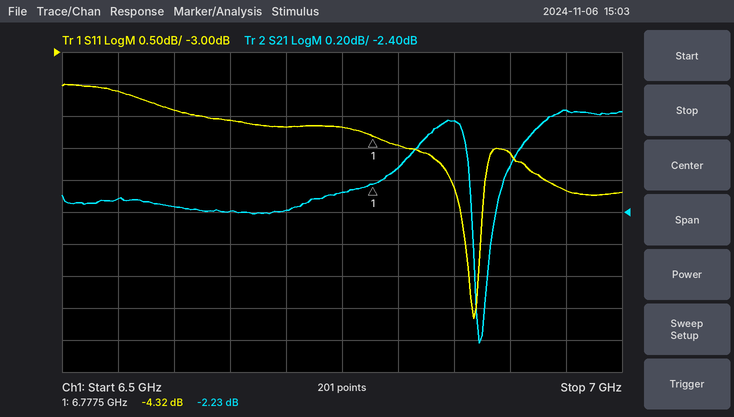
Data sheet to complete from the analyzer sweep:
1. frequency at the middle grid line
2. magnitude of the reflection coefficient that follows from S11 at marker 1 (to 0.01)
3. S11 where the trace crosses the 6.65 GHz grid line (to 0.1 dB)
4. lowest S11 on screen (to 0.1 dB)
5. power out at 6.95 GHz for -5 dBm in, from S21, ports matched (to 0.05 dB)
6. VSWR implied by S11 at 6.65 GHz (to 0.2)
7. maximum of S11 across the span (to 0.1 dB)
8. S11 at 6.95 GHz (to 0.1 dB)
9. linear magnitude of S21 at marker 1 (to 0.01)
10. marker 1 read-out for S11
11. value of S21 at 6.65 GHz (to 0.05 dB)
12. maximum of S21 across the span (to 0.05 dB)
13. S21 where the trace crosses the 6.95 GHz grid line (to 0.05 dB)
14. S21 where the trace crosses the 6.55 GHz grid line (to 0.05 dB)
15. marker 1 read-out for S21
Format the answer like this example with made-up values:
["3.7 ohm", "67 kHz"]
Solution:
["6.75 GHz", "0.61", "-4.1 dB", "-7.2 dB", "-6.75 dBm", "4.4", "-3.5 dB", "-5.2 dB", "0.77", "-4.32 dB", "-2.40 dB", "-1.75 dB", "-1.75 dB", "-2.30 dB", "-2.23 dB"]
